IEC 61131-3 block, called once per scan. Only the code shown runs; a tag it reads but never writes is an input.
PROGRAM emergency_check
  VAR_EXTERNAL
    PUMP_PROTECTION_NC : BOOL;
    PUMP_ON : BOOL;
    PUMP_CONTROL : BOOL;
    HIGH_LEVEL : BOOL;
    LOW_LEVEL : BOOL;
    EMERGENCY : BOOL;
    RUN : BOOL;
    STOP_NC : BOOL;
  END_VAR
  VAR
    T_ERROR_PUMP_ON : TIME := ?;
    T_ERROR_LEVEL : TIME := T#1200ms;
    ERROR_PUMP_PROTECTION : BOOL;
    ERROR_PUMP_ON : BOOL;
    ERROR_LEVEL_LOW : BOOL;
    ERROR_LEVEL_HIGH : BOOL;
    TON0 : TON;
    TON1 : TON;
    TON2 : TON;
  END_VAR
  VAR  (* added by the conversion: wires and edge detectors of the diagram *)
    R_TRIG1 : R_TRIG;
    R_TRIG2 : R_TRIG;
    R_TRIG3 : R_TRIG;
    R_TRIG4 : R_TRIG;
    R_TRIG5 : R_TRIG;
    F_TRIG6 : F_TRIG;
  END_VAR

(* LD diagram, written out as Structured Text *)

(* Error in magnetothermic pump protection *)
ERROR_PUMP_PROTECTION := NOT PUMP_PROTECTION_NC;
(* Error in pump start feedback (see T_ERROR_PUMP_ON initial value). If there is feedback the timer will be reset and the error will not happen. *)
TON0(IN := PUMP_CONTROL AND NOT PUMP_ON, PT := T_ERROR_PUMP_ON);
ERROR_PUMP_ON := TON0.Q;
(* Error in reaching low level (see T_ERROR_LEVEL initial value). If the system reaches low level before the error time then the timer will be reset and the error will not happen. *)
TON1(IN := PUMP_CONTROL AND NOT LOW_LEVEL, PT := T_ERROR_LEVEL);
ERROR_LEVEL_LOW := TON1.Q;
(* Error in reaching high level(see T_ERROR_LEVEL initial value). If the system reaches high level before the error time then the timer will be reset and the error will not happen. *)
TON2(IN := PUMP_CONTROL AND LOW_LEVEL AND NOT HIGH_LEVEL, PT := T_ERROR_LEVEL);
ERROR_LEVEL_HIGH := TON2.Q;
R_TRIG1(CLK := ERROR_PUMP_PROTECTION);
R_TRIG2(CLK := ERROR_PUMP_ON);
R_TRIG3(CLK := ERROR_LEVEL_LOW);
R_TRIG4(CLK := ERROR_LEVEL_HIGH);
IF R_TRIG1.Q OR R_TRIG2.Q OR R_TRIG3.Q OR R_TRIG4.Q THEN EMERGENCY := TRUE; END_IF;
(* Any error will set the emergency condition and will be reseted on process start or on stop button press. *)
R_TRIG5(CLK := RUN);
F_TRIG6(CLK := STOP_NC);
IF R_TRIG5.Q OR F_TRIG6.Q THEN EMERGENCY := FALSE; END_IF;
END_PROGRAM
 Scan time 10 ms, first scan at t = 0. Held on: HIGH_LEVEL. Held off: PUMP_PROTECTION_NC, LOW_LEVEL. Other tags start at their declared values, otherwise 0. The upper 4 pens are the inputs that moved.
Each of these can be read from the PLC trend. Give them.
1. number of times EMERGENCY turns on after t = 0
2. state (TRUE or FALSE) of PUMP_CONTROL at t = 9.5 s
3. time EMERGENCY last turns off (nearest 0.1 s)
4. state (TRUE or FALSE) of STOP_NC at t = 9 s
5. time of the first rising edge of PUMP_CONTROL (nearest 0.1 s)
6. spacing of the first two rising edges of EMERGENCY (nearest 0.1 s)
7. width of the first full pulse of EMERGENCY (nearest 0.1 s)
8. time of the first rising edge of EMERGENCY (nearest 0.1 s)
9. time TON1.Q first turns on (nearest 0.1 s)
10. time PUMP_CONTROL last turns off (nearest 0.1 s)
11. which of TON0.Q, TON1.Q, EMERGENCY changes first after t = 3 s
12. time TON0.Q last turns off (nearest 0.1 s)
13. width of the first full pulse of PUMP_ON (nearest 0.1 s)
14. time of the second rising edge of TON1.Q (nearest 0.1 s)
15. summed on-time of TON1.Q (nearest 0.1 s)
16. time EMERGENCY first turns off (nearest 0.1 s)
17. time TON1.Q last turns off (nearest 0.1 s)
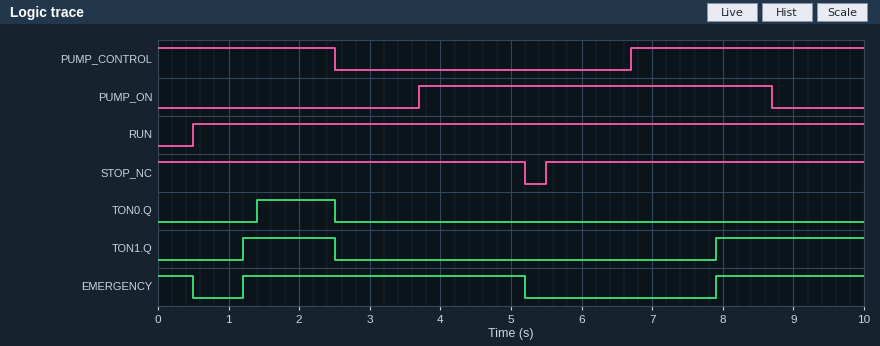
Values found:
2
TRUE
5.2 s
TRUE
6.7 s
6.7 s
4.0 s
1.2 s
1.2 s
2.5 s
EMERGENCY
2.5 s
5.0 s
7.9 s
3.4 s
0.5 s
2.5 s
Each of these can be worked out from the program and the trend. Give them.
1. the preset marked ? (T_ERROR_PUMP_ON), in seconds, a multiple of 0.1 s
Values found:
1.4 s
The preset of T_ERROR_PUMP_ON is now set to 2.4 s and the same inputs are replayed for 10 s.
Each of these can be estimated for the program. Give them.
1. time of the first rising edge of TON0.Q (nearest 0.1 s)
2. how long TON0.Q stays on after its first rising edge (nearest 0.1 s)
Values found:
2.4 s
0.1 s
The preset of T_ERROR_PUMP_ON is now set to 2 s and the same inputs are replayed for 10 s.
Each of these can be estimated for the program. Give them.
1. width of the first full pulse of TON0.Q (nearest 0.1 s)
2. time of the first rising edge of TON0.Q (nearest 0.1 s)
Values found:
0.5 s
2.0 s
